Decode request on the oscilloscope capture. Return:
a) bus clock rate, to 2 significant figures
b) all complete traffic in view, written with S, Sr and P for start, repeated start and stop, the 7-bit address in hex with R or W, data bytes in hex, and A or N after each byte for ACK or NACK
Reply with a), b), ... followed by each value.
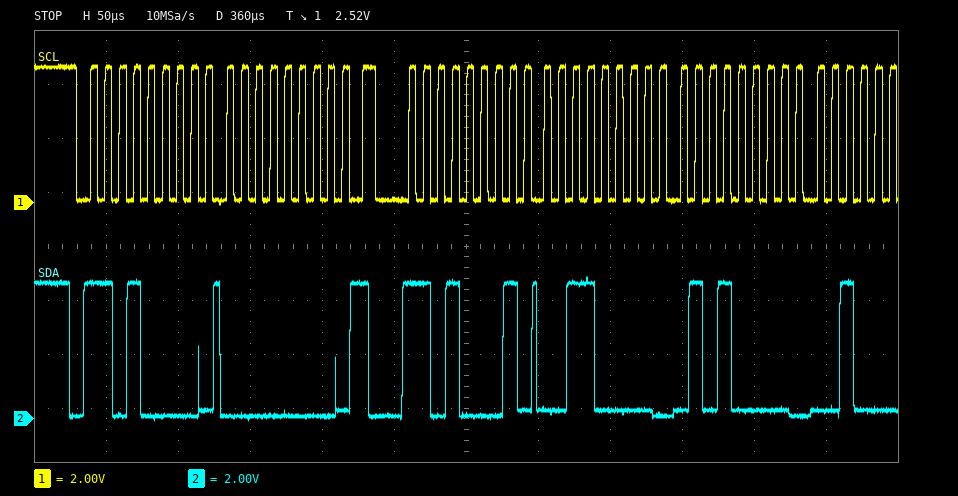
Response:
a) 100 kHz
b) S 68W A 00 A Sr 68R A 30 A 50 A
